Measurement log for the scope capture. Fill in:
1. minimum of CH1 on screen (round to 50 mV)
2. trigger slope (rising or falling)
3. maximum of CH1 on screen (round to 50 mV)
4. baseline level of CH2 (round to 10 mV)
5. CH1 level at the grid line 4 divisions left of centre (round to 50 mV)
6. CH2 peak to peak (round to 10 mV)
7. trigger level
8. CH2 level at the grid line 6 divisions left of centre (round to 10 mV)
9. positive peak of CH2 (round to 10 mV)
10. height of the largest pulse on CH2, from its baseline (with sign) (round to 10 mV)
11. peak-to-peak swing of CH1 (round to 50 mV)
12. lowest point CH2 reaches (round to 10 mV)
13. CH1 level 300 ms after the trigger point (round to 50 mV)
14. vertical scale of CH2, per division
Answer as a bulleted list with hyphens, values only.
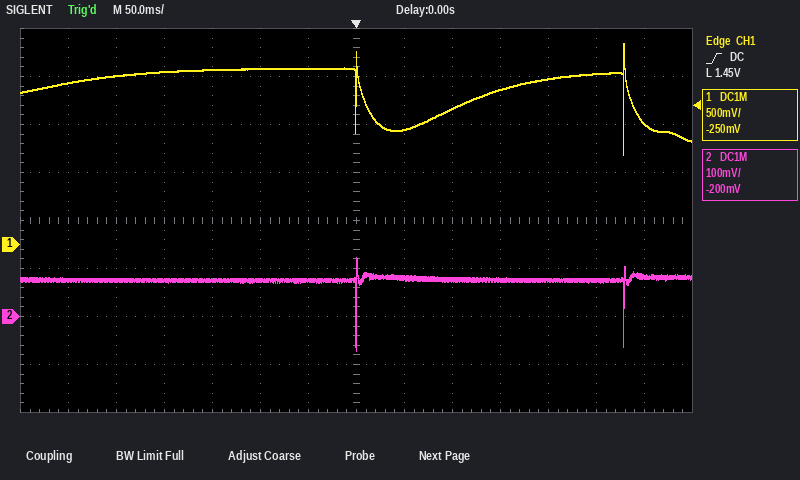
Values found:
- 950 mV
- rising
- 2.10 V
- 80 mV
- 1.80 V
- 190 mV
- 1.45 V
- 80 mV
- 120 mV
- -150 mV
- 1.15 V
- -70 mV
- 1.25 V
- 100 mV
